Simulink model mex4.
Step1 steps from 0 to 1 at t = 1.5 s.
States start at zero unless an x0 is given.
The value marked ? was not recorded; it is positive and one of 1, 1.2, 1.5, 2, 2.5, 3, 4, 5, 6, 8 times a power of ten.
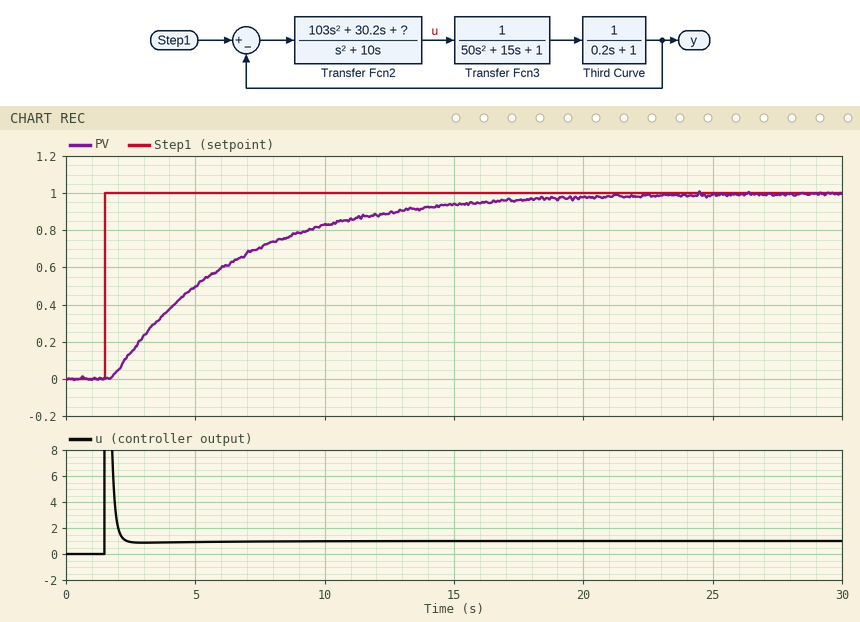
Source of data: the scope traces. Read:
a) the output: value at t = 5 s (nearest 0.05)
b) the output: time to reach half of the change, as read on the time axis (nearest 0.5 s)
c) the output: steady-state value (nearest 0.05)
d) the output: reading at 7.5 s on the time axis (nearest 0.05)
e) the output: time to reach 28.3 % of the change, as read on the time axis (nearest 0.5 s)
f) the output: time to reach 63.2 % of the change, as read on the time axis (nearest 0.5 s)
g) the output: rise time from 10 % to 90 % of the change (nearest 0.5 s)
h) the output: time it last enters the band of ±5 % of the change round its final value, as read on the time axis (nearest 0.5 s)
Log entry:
0.50
5.0 s
1.00
0.70
3.5 s
6.5 s
10.5 s
16.0 s
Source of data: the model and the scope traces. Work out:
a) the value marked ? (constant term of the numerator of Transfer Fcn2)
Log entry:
2
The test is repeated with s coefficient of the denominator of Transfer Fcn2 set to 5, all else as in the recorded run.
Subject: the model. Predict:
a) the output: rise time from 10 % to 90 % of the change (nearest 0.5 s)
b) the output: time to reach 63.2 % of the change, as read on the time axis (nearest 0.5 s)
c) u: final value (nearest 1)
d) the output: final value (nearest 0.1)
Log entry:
4.5 s
4.0 s
1
1.0
